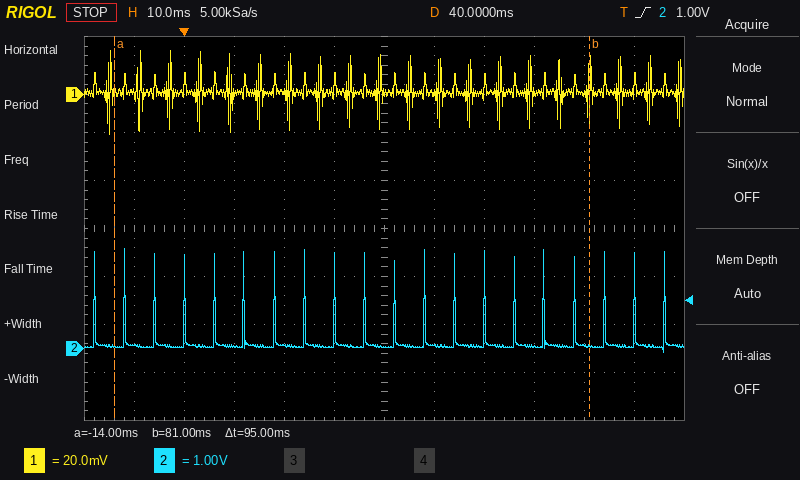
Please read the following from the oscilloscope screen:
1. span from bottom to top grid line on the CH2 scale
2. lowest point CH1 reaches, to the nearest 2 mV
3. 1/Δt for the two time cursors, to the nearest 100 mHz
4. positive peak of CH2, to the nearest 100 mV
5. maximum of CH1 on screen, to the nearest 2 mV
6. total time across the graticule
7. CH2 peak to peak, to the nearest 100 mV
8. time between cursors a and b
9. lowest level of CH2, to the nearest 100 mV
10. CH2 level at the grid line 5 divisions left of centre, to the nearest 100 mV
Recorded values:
8 V
-16 mV
10.5 Hz
2.1 V
18 mV
120 ms
2.2 V
95 ms
-100 mV
100 mV
